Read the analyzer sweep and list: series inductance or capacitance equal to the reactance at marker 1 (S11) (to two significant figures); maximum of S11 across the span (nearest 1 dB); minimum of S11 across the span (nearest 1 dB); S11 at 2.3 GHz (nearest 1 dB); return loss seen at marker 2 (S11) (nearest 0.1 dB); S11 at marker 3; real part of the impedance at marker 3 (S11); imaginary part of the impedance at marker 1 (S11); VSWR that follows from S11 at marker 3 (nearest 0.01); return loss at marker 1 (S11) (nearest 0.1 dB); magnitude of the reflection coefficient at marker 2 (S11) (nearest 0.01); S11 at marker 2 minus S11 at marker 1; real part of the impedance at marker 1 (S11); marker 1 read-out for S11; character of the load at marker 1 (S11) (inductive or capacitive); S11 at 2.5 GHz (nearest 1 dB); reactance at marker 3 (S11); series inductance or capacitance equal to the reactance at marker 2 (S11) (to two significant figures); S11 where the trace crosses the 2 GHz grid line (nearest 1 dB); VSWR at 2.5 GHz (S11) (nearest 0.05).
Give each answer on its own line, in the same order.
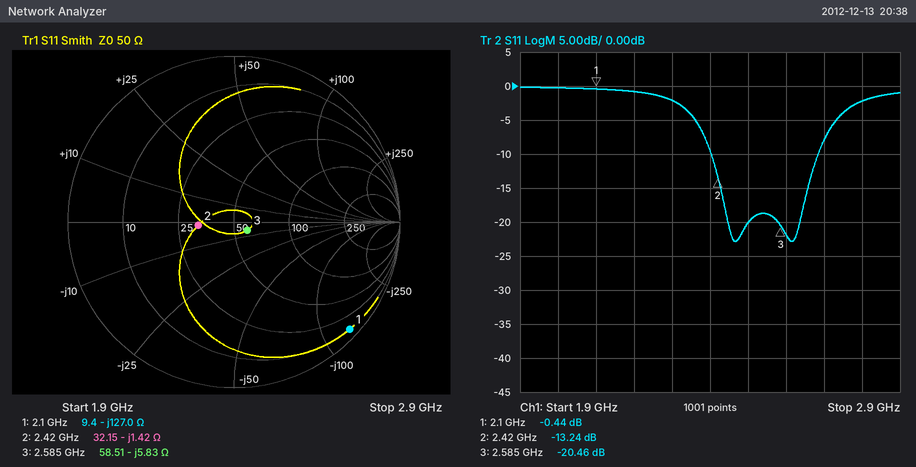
600 fF
0 dB
-23 dB
-2 dB
13.2 dB
-20.46 dB
58.51 Ω
-127.0 Ω
1.21
0.4 dB
0.22
-12.80 dB
9.4 Ω
-0.44 dB
capacitive
-20 dB
-5.83 Ω
46 pF
0 dB
1.20
